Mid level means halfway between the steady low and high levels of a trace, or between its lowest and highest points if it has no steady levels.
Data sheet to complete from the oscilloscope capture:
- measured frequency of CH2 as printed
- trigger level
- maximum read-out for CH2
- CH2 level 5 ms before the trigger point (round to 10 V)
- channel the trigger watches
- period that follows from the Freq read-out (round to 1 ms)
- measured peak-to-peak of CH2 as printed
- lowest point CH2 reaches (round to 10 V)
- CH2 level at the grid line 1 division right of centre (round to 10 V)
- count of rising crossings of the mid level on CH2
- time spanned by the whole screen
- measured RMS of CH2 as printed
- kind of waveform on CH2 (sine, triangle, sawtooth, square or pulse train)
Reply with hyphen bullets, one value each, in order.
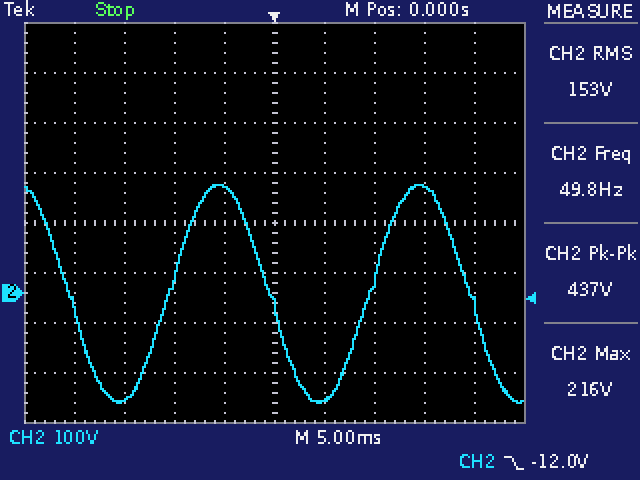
- 49.8 Hz
- -12.0 V
- 216 V
- 210 V
- CH2
- 20 ms
- 437 V
- -220 V
- -210 V
- 2
- 50 ms
- 153 V
- sine
